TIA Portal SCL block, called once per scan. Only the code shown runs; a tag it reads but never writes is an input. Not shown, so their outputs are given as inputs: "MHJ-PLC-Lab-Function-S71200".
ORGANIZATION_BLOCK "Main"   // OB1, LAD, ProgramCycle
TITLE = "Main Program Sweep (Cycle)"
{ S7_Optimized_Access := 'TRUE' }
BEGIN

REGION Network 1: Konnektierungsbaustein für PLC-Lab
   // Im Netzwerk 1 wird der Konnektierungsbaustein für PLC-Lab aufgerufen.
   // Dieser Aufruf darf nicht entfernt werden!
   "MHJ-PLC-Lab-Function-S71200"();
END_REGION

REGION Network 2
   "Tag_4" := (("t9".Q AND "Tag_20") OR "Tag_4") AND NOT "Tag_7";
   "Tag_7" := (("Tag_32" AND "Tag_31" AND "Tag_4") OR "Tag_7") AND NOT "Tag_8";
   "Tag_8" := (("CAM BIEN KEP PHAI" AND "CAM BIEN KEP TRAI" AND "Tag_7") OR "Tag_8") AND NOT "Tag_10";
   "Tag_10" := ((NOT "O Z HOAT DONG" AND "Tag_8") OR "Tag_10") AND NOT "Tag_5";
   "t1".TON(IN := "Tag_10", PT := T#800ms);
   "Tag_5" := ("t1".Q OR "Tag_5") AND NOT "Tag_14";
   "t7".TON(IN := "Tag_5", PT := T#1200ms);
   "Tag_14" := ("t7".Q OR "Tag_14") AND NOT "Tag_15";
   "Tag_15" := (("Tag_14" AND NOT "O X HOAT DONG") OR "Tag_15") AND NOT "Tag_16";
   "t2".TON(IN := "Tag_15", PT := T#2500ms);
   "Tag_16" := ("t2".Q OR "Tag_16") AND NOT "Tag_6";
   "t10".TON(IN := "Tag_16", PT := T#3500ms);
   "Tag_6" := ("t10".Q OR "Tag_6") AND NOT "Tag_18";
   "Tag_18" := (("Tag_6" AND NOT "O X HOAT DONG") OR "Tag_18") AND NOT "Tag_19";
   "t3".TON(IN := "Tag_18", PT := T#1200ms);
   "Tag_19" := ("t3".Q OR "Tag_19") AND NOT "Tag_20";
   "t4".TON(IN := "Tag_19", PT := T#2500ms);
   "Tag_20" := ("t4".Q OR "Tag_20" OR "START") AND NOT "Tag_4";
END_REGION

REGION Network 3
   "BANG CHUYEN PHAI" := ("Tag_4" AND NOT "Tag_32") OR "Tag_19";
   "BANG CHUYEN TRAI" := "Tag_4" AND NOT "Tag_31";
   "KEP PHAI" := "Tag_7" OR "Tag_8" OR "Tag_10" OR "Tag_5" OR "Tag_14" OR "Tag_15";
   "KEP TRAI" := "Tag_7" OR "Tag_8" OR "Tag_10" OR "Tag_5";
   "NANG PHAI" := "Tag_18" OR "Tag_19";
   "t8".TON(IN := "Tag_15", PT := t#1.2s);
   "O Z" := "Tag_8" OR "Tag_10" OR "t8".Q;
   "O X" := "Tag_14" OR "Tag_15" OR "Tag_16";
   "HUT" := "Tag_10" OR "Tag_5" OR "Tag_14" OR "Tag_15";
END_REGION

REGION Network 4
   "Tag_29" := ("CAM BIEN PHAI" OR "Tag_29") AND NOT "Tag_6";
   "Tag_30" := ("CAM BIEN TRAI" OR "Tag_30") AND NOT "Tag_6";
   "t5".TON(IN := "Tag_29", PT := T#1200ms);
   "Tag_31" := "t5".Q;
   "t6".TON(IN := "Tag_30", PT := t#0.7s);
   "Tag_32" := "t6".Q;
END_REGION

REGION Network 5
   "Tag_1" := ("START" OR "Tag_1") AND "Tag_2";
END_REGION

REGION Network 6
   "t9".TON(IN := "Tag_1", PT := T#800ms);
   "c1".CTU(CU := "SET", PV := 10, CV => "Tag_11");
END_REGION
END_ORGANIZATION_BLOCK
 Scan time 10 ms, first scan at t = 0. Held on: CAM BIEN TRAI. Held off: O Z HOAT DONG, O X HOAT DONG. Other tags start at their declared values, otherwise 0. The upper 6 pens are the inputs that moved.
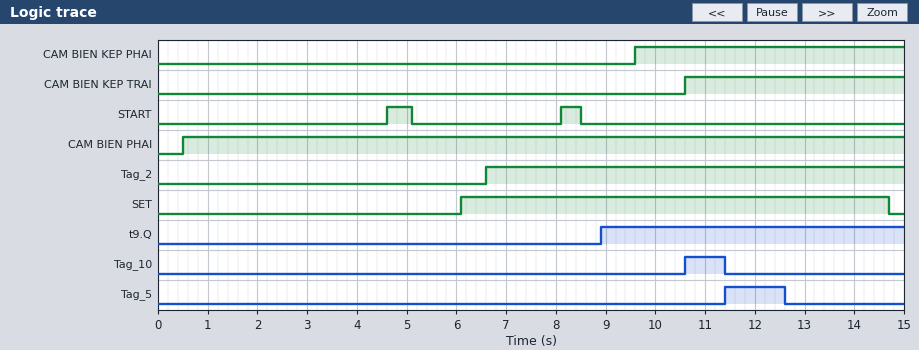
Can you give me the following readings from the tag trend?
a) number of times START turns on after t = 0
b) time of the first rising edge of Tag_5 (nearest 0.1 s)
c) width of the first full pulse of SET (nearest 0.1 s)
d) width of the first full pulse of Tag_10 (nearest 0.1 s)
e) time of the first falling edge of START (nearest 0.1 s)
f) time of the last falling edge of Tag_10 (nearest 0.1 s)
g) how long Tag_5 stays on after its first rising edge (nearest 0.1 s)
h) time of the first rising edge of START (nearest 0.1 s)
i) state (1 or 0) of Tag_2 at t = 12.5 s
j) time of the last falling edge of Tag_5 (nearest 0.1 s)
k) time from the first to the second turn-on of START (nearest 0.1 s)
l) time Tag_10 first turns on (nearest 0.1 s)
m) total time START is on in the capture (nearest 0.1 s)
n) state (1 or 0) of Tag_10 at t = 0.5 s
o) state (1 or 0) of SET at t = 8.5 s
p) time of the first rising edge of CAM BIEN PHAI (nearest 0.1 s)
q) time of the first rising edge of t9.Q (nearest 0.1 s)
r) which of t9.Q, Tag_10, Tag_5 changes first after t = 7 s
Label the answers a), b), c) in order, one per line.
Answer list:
a) 2
b) 11.4 s
c) 8.6 s
d) 0.8 s
e) 5.1 s
f) 11.4 s
g) 1.2 s
h) 4.6 s
i) 1
j) 12.6 s
k) 3.5 s
l) 10.6 s
m) 0.9 s
n) 0
o) 1
p) 0.5 s
q) 8.9 s
r) t9.Q
